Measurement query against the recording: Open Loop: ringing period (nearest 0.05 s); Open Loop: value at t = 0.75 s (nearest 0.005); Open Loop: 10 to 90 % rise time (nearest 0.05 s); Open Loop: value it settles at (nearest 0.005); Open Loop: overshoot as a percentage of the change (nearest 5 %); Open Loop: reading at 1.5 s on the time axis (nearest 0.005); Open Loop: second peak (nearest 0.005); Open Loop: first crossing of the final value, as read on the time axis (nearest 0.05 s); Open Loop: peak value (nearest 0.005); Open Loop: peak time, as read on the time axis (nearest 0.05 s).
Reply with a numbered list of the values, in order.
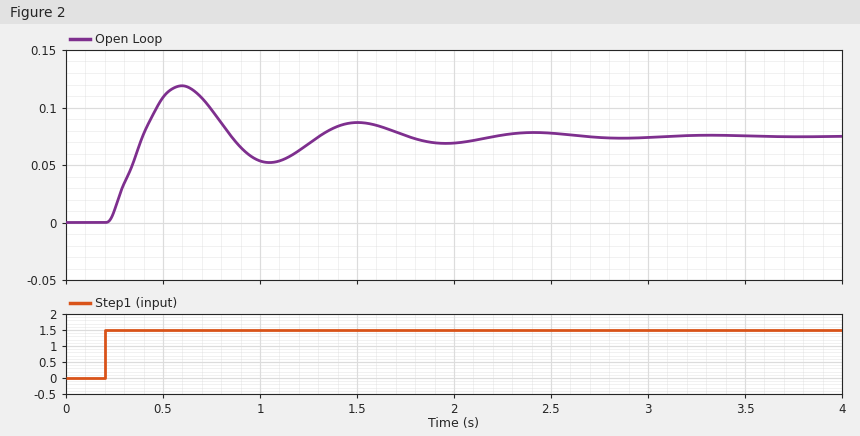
1. 0.90 s
2. 0.100
3. 0.15 s
4. 0.075
5. 60 %
6. 0.085
7. 0.085
8. 0.40 s
9. 0.120
10. 0.60 s
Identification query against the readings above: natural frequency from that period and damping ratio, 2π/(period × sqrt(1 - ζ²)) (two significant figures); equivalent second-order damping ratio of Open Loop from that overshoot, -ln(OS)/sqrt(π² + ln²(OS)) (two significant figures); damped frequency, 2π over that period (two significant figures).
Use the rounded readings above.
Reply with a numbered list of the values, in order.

1. 7.1 rad/s
2. 0.16
3. 7.0 rad/s
